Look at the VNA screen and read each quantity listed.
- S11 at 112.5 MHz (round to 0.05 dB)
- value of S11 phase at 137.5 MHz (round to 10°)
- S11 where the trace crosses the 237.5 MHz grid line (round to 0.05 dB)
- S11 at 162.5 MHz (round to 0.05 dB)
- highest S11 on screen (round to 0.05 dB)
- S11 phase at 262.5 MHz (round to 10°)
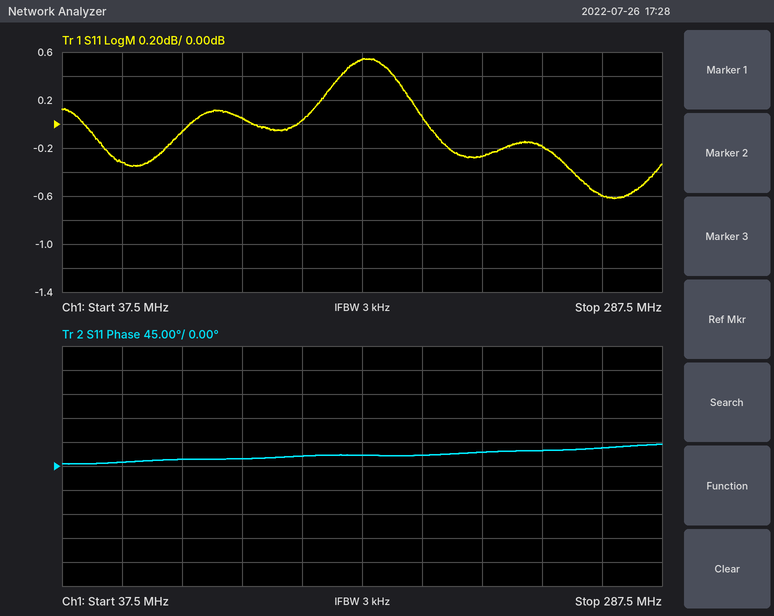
0.05 dB
20°
-0.20 dB
0.55 dB
0.55 dB
30°
